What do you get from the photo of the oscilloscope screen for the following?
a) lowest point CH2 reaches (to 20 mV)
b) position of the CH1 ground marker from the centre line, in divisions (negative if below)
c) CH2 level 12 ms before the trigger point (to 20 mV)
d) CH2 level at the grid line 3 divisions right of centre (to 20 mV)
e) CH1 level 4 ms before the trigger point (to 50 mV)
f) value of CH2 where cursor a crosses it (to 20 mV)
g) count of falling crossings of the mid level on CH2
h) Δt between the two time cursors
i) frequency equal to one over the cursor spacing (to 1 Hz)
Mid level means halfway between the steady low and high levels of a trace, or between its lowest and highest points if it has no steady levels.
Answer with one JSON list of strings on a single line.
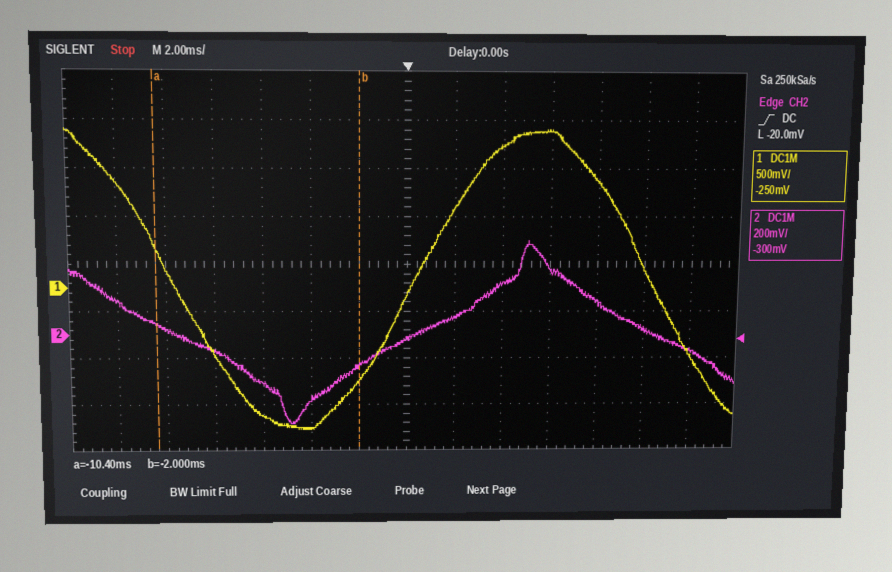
["-380 mV", "-0.5 div", "140 mV", "280 mV", "-1.50 V", "40 mV", "2", "8.4 ms", "119 Hz"]
